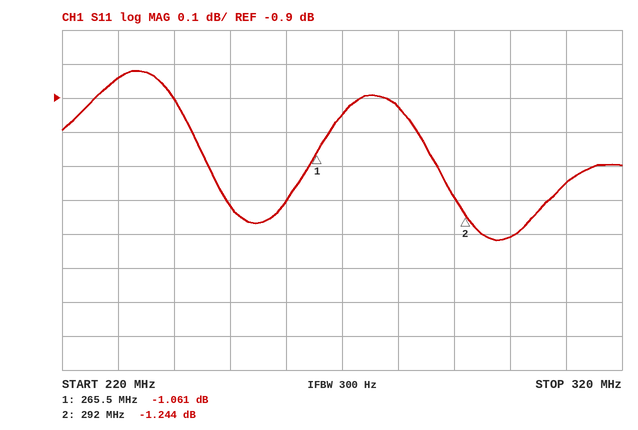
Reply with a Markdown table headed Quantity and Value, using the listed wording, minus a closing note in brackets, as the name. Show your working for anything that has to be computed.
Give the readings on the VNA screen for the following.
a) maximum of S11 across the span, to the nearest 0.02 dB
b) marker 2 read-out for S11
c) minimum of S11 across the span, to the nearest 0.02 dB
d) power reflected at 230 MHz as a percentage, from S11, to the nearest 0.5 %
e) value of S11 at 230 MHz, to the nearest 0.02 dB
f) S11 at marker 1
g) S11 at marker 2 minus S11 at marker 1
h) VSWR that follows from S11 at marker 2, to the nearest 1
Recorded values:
| Quantity | Value |
|---|---|
| maximum of S11 across the span, to the nearest 0.02 dB | -0.82 dB |
| marker 2 read-out for S11 | -1.244 dB |
| minimum of S11 across the span, to the nearest 0.02 dB | -1.32 dB |
| power reflected at 230 MHz as a percentage, from S11, to the nearest 0.5 % | 10^(-0.84/10) ≈ 82.4 %, so 82.5 % to the nearest 0.5 % |
| value of S11 at 230 MHz, to the nearest 0.02 dB | -0.84 dB |
| S11 at marker 1 | -1.061 dB |
| S11 at marker 2 minus S11 at marker 1 | -1.244 − (-1.061) = -0.183 dB |
| VSWR that follows from S11 at marker 2, to the nearest 1 | (1 + 0.8666)/(1 − 0.8666) ≈ 14 |
